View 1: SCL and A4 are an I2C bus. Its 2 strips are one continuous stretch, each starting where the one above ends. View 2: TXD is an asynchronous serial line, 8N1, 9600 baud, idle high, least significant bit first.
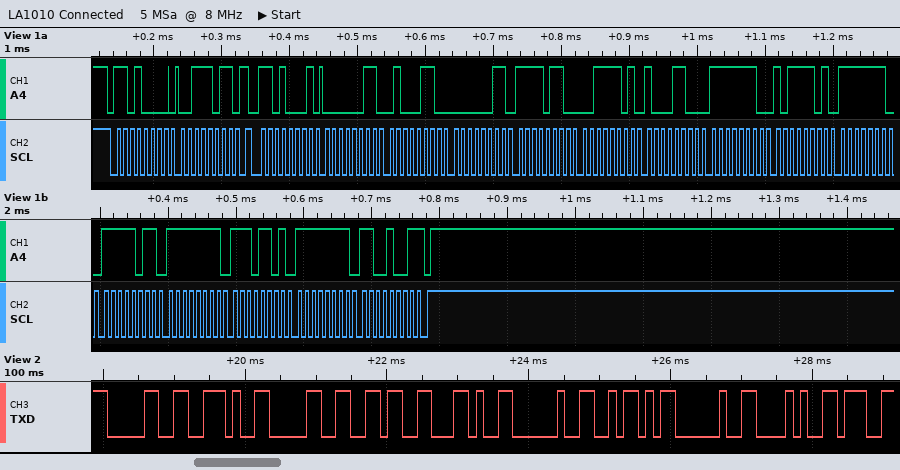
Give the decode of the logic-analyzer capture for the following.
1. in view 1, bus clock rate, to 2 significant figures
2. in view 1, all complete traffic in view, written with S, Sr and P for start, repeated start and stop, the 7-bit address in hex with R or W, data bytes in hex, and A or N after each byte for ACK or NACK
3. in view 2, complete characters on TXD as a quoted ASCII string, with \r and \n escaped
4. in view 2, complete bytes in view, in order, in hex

100 kHz
S 68W A 3B A Sr 68R A 03 A 46 A 03 A F6 A 3D A 8C A FE A BD A FE A FB A FF A ED A FF A C9 N P
"0.06, Z ("
30 2E 30 36 2C 20 5A 20 28
